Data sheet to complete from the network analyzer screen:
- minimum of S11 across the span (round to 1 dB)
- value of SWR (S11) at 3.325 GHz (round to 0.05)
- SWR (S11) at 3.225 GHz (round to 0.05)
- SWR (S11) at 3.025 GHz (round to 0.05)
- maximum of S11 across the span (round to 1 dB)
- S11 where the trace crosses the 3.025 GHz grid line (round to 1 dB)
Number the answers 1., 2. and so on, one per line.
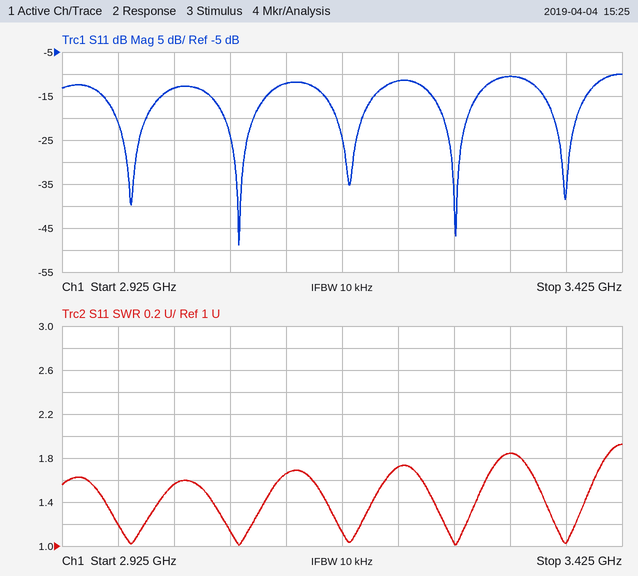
1. -49 dB
2. 1.85
3. 1.70
4. 1.55
5. -10 dB
6. -13 dB
